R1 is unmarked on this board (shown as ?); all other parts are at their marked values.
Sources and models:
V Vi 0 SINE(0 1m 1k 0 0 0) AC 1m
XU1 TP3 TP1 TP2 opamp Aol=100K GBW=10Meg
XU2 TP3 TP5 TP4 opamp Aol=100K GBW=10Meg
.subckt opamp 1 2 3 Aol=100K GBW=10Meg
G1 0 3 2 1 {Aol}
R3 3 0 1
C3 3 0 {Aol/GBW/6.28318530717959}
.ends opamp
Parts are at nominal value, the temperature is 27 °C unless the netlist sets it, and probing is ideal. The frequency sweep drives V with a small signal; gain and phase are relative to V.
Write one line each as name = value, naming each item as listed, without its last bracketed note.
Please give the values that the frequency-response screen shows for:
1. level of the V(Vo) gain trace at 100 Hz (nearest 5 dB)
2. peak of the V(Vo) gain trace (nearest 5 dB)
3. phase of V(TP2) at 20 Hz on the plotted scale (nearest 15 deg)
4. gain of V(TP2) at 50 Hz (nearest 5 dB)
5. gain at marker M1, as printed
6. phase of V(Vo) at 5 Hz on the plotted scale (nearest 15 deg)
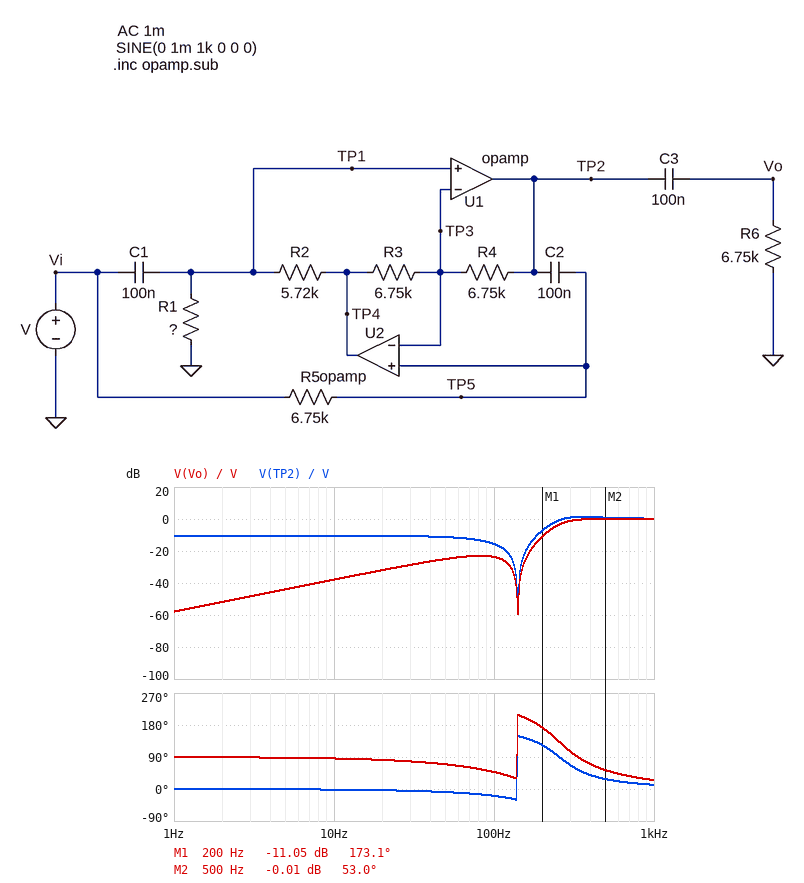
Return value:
level of the V(Vo) gain trace at 100 Hz = -25 dB
peak of the V(Vo) gain trace = 0 dB
phase of V(TP2) at 20 Hz on the plotted scale = 0 deg
gain of V(TP2) at 50 Hz = -10 dB
gain at marker M1, as printed = -11.05 dB
phase of V(Vo) at 5 Hz on the plotted scale = 90 deg
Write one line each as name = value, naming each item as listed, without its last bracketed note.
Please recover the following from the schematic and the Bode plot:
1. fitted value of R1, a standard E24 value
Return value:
fitted value of R1, a standard E24 value = 8.2 kΩ
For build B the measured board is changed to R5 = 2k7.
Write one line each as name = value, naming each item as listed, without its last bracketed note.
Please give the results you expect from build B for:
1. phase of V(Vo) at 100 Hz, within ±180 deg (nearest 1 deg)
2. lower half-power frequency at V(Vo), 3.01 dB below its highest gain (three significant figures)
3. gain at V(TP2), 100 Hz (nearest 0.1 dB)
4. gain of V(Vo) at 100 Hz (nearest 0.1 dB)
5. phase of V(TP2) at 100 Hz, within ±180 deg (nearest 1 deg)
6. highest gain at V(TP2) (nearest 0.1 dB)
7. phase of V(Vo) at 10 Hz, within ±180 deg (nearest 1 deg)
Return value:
phase of V(Vo) at 100 Hz, within ±180 deg = 60 deg
lower half-power frequency at V(Vo), 3.01 dB below its highest gain = 375 Hz
gain at V(TP2), 100 Hz = -11.9 dB
gain of V(Vo) at 100 Hz = -20.0 dB
phase of V(TP2) at 100 Hz, within ±180 deg = -7 deg
highest gain at V(TP2) = 4.1 dB
phase of V(Vo) at 10 Hz, within ±180 deg = 87 deg
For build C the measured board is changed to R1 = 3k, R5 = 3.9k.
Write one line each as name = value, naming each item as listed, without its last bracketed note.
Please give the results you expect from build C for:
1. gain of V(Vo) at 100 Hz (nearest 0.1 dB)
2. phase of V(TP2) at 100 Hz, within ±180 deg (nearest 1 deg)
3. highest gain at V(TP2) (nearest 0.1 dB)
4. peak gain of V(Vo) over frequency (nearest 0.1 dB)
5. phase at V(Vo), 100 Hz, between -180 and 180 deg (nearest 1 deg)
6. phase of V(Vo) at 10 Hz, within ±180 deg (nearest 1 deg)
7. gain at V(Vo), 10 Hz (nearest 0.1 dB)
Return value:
gain of V(Vo) at 100 Hz = -8.4 dB
phase of V(TP2) at 100 Hz, within ±180 deg = 153 deg
highest gain at V(TP2) = 1.7 dB
peak gain of V(Vo) over frequency = 0.6 dB
phase at V(Vo), 100 Hz, between -180 and 180 deg = -140 deg
phase of V(Vo) at 10 Hz, within ±180 deg = -95 deg
gain at V(Vo), 10 Hz = -28.3 dB
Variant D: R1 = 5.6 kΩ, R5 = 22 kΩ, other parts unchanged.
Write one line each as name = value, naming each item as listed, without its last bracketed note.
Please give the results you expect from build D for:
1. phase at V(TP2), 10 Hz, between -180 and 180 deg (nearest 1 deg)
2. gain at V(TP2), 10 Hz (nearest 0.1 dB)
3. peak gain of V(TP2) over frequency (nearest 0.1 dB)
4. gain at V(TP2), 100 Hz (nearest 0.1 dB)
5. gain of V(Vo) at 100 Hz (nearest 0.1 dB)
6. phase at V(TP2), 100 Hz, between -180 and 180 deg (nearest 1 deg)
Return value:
phase at V(TP2), 10 Hz, between -180 and 180 deg = 172 deg
gain at V(TP2), 10 Hz = -31.6 dB
peak gain of V(TP2) over frequency = 0 dB
gain at V(TP2), 100 Hz = -9.2 dB
gain of V(Vo) at 100 Hz = -17.4 dB
phase at V(TP2), 100 Hz, between -180 and 180 deg = 110 deg
